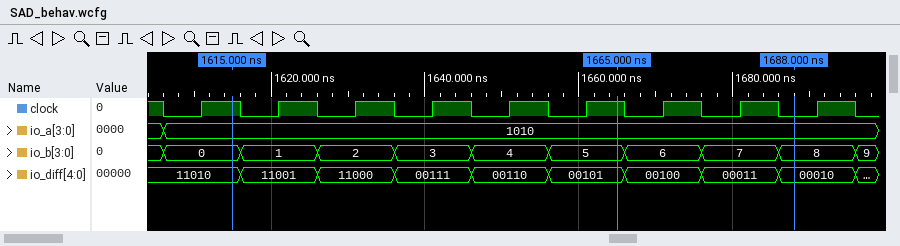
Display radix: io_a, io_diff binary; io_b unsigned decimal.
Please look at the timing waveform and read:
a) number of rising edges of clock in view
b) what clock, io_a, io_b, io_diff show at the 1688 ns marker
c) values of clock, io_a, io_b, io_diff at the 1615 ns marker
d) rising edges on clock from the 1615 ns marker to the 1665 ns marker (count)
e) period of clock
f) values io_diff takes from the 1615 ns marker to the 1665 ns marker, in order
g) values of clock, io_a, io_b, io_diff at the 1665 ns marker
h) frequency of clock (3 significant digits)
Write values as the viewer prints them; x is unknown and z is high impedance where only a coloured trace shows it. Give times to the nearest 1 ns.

9
clock=0, io_a=1010, io_b=8, io_diff=00010
clock=1, io_a=1010, io_b=0, io_diff=11010
5
10 ns
11010, 11001, 11000, 00111, 00110, 00101
clock=1, io_a=1010, io_b=5, io_diff=00101
100 MHz
